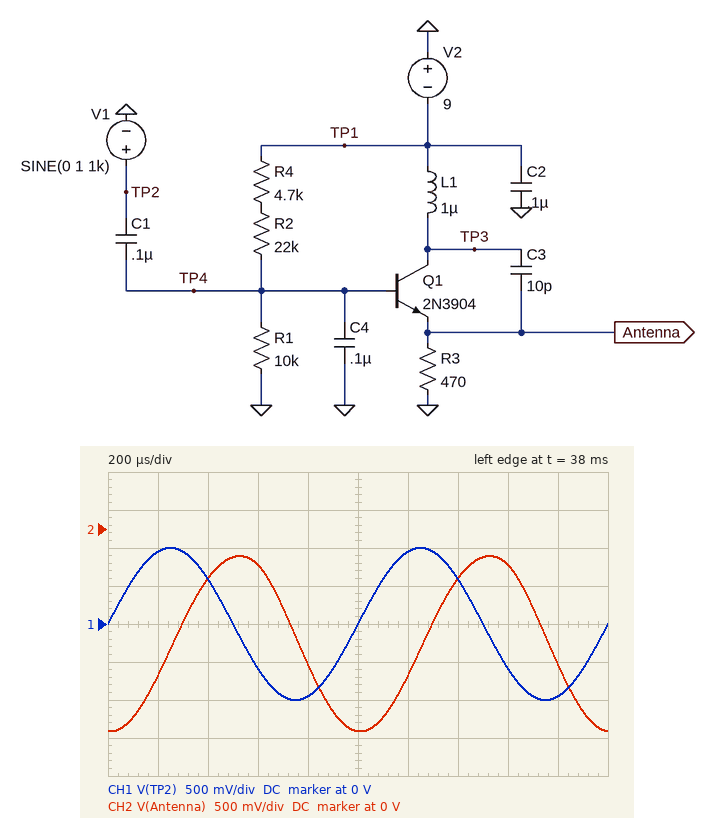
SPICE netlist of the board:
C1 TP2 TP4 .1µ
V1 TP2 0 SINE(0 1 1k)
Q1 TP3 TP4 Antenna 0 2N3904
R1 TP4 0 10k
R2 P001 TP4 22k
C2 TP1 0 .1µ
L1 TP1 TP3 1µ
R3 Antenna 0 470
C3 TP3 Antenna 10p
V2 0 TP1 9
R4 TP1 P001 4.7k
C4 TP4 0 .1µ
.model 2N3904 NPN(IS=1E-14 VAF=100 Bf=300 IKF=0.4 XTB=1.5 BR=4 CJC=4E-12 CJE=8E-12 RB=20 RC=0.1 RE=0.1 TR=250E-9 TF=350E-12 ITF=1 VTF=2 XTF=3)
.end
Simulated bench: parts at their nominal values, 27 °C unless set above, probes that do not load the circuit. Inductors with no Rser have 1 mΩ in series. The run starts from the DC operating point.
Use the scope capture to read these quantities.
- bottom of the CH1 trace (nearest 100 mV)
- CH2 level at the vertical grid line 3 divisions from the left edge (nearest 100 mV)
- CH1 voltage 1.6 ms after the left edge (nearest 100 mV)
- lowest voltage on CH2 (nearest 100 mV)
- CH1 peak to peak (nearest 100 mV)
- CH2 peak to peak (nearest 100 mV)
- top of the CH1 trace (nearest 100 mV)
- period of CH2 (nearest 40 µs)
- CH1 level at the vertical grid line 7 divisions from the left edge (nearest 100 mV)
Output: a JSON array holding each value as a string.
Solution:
["-1.0 V", "-500 mV", "-600 mV", "-2.7 V", "2.0 V", "2.3 V", "1.0 V", "1.00 ms", "600 mV"]
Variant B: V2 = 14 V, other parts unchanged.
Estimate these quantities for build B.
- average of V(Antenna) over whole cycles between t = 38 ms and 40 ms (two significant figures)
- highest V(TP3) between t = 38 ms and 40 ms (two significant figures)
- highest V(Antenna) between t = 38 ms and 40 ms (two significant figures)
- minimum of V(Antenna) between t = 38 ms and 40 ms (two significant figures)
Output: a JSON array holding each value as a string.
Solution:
["-2.4 V", "-14 V", "-1.3 V", "-3.6 V"]
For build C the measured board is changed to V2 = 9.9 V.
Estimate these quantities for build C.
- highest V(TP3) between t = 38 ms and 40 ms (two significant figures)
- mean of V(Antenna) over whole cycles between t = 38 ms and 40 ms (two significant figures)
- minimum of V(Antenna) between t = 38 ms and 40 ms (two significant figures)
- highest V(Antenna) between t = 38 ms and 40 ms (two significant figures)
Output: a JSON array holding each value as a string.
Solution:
["-9.9 V", "-1.7 V", "-2.8 V", "-520 mV"]
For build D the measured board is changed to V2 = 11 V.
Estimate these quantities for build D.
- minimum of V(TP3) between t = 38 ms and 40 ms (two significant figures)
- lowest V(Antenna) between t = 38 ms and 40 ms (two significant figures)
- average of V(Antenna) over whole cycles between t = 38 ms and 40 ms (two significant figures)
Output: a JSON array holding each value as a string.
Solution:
["-11 V", "-3.0 V", "-1.9 V"]
